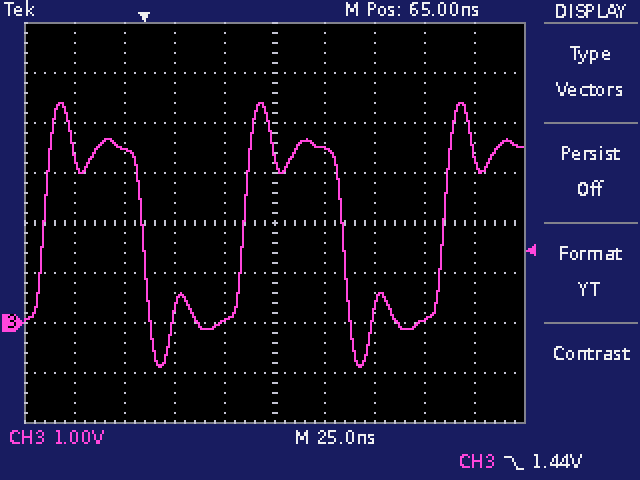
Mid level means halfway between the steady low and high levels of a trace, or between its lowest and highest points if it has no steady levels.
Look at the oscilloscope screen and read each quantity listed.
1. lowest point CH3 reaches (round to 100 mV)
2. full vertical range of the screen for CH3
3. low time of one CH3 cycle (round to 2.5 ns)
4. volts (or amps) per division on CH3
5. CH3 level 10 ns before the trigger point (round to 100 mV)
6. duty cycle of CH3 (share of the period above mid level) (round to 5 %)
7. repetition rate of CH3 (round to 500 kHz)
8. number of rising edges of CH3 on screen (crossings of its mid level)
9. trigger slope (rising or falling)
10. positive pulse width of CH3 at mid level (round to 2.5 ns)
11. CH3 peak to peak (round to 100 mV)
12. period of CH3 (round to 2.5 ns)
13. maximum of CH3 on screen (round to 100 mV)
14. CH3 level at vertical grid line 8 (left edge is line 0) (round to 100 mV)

-900 mV
8 V
50.0 ns
1 V
3.5 V
50 %
10.0 MHz
3
falling
50.0 ns
5.3 V
100.0 ns
4.4 V
100 mV
